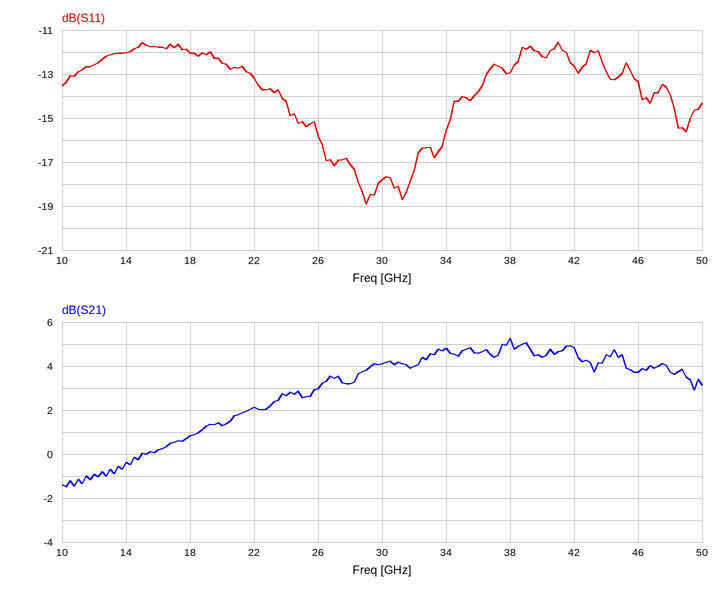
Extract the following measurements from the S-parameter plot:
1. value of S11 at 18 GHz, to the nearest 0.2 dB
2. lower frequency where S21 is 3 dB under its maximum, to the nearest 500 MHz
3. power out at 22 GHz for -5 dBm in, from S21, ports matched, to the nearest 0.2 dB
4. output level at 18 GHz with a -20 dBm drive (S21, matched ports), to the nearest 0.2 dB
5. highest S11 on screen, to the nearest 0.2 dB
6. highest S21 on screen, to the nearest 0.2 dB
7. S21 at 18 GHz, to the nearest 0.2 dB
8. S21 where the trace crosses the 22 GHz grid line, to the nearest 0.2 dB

-12.0 dB
23.0 GHz
-2.8 dBm
-19.2 dBm
-11.6 dB
5.2 dB
0.8 dB
2.2 dB
